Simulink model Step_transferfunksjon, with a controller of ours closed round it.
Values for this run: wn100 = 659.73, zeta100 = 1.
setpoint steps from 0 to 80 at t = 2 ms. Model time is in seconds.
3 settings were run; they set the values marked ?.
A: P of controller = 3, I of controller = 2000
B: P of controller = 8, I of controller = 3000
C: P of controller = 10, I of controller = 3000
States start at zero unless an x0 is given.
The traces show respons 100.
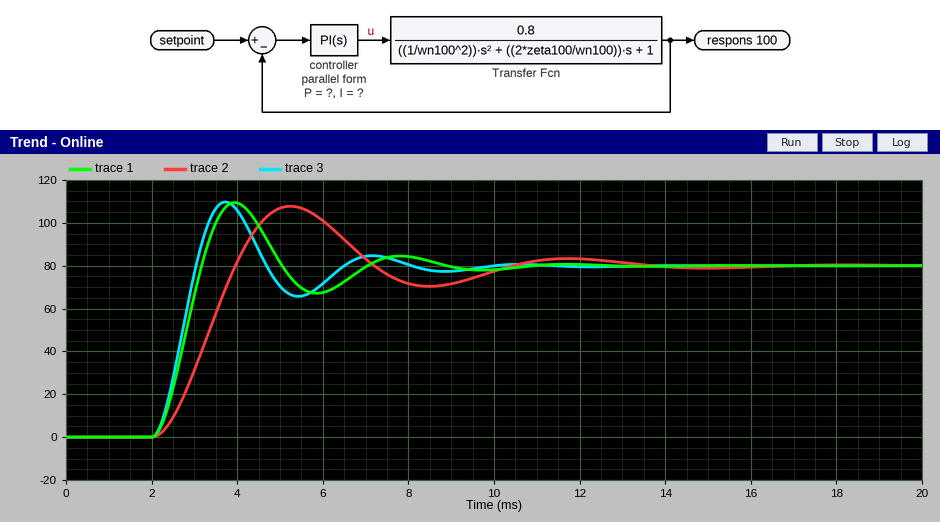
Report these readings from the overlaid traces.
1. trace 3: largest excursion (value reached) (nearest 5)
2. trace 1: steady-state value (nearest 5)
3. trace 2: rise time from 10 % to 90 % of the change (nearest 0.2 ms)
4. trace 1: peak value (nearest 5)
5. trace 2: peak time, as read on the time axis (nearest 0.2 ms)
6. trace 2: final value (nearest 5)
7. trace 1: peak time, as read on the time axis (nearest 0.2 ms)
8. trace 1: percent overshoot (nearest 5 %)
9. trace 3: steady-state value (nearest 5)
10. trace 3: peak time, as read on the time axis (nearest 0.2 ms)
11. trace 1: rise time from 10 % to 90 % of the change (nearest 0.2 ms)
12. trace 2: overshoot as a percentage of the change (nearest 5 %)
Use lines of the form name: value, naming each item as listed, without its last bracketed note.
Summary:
trace 3: largest excursion (value reached): 110
trace 1: steady-state value: 80
trace 2: rise time from 10 % to 90 % of the change: 1.4 ms
trace 1: peak value: 110
trace 2: peak time, as read on the time axis: 5.2 ms
trace 2: final value: 80
trace 1: peak time, as read on the time axis: 4.0 ms
trace 1: percent overshoot: 35 %
trace 3: steady-state value: 80
trace 3: peak time, as read on the time axis: 3.8 ms
trace 1: rise time from 10 % to 90 % of the change: 0.8 ms
trace 2: overshoot as a percentage of the change: 35 %
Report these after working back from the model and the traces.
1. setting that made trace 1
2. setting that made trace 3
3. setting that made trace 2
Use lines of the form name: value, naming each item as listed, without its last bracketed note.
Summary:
setting that made trace 1: B
setting that made trace 3: C
setting that made trace 2: A
